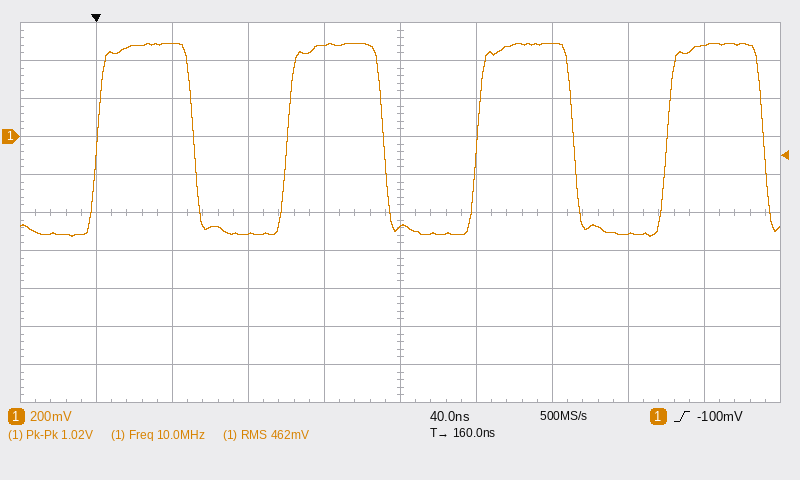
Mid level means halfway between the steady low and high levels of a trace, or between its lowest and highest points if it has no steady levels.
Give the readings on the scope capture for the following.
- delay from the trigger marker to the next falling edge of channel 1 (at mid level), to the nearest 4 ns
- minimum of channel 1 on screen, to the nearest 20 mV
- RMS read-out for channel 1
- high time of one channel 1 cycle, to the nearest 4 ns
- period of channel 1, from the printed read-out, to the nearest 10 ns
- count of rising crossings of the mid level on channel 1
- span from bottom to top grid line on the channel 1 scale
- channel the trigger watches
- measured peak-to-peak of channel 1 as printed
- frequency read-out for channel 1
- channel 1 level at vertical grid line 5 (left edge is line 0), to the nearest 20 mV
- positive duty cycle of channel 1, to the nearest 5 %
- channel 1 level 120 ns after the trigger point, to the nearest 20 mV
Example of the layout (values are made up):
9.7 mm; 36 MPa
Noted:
52 ns; -520 mV; 462 mV; 52 ns; 100 ns; 4; 2 V; channel 1; 1.02 V; 10.0 MHz; -480 mV; 50 %; 480 mV
